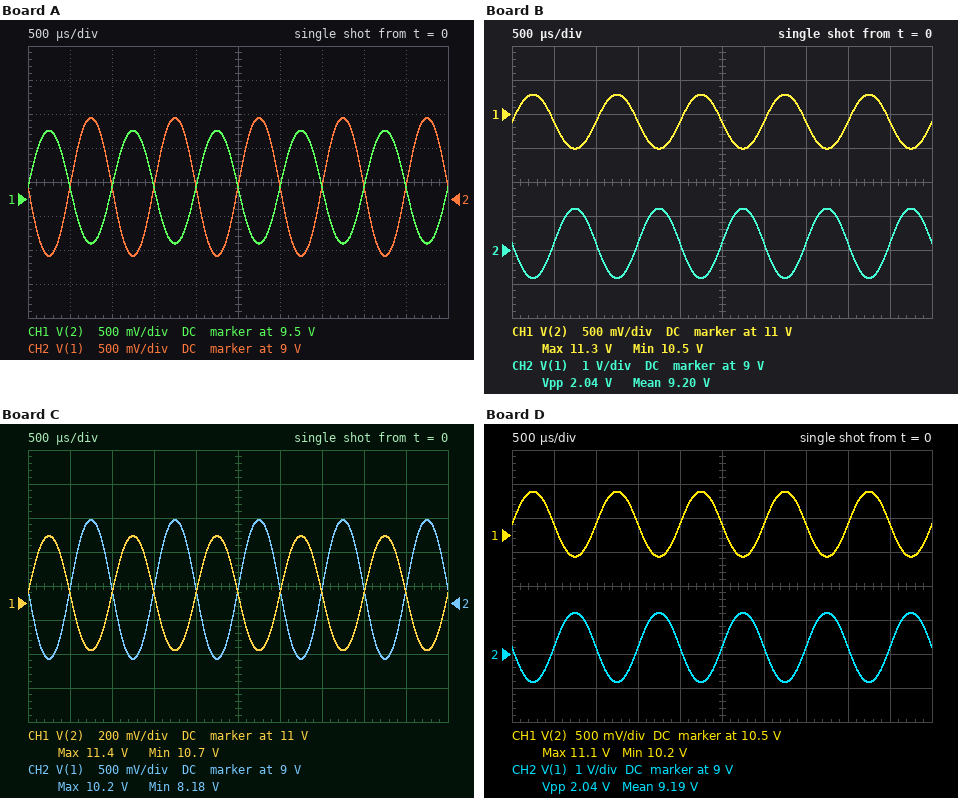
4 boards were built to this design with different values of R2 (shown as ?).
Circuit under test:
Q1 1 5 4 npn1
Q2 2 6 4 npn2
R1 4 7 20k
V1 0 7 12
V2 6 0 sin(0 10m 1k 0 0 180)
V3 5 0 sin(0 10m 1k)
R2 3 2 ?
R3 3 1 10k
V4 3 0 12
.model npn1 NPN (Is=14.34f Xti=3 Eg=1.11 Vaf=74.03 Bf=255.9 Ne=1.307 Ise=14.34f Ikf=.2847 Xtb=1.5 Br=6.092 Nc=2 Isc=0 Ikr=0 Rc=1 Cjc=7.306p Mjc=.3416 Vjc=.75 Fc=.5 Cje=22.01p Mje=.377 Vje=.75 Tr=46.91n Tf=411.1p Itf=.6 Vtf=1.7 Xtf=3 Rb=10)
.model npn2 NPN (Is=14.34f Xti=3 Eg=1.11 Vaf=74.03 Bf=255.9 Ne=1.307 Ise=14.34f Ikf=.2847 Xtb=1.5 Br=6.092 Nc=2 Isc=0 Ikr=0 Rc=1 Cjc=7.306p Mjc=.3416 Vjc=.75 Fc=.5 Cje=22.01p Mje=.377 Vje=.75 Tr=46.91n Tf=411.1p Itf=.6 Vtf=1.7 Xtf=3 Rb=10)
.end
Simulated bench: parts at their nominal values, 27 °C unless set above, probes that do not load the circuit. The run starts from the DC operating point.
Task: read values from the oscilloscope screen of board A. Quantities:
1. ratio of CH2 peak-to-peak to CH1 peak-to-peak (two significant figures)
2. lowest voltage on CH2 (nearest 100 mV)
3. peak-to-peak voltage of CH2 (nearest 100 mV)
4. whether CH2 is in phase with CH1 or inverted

1.2
8.2 V
2.0 V
inverted
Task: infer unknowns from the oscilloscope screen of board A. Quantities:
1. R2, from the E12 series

8.2 kΩ
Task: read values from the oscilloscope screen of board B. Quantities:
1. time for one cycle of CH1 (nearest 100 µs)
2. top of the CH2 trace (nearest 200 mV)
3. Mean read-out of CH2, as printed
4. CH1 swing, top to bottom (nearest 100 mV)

1.0 ms
10.2 V
9.20 V
800 mV
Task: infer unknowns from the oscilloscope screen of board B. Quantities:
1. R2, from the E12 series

3.9 kΩ
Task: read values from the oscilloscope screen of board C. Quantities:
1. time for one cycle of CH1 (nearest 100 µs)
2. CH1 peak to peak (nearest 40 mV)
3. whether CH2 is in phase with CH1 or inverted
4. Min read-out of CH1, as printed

1.0 ms
680 mV
inverted
10.7 V
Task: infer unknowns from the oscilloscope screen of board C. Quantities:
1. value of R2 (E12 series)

3.3 kΩ
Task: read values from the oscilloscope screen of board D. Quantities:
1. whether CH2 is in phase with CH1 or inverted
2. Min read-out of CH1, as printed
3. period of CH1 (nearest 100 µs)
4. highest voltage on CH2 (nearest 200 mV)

inverted
10.2 V
1.0 ms
10.2 V
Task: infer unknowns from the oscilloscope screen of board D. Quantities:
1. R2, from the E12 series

4.7 kΩ
